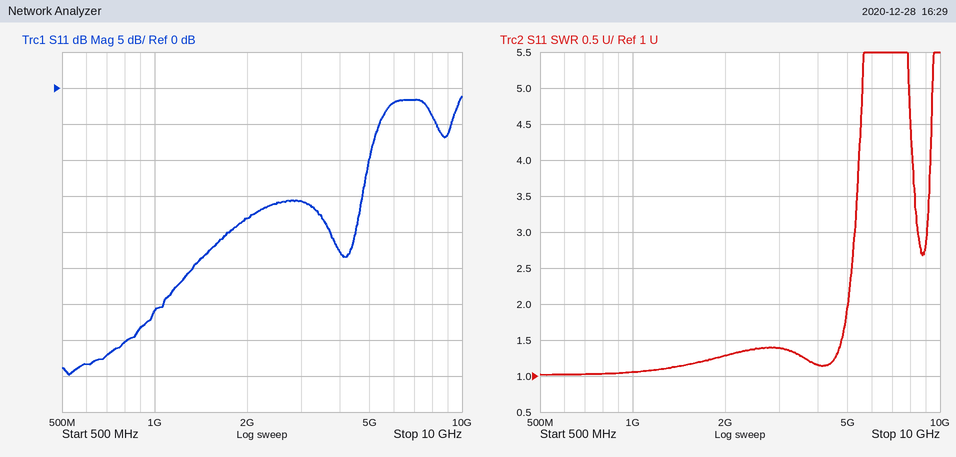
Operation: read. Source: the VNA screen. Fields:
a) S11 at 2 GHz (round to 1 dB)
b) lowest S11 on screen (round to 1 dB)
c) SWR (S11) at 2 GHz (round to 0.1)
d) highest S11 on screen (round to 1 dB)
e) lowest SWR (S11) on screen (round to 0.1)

-18 dB
-40 dB
1.3
-1 dB
1.0
